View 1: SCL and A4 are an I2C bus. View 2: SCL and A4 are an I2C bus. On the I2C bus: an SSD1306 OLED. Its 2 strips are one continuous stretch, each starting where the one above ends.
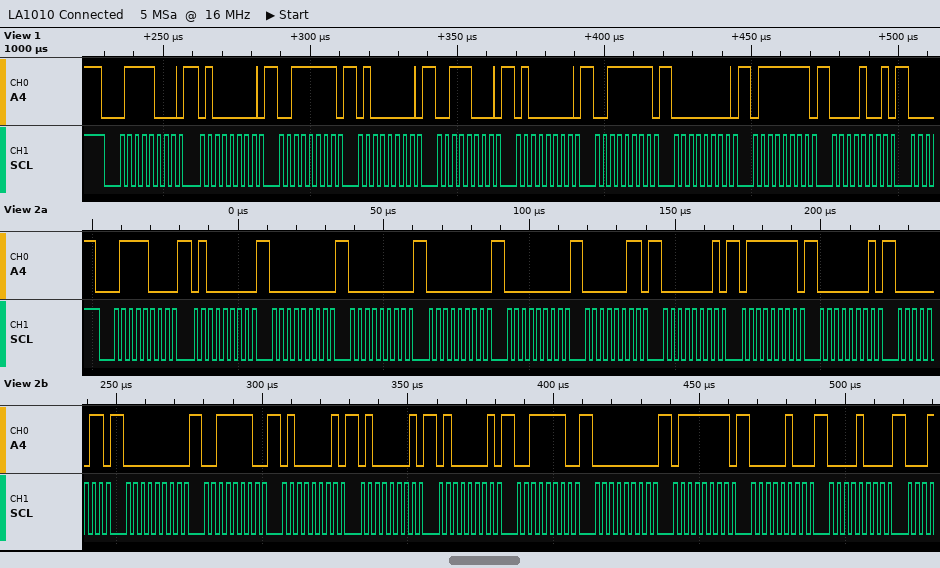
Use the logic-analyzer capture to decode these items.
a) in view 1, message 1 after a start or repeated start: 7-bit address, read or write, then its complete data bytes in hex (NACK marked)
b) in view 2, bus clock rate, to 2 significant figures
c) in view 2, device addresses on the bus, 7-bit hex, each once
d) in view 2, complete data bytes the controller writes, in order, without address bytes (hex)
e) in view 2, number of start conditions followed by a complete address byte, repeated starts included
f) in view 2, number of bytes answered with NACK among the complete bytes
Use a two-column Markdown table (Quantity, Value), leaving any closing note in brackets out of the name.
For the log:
| Quantity | Value |
|---|---|
| in view 1, message 1 after a start or repeated start: 7-bit address, read or write, then its complete data bytes in hex | 0x3C write: 40 3F 40 38 40 3F 00 7F 09 |
| in view 2, bus clock rate, to 2 significant figures | 400 kHz |
| in view 2, device addresses on the bus, 7-bit hex, each once | 0x3C |
| in view 2, complete data bytes the controller writes, in order, without address bytes | 40 00 00 00 00 03 01 7F 01 03 00 3E 41 41 41 3E 00 7F 04 08 |
| in view 2, number of start conditions followed by a complete address byte, repeated starts included | 1 |
| in view 2, number of bytes answered with NACK among the complete bytes | 0 |
